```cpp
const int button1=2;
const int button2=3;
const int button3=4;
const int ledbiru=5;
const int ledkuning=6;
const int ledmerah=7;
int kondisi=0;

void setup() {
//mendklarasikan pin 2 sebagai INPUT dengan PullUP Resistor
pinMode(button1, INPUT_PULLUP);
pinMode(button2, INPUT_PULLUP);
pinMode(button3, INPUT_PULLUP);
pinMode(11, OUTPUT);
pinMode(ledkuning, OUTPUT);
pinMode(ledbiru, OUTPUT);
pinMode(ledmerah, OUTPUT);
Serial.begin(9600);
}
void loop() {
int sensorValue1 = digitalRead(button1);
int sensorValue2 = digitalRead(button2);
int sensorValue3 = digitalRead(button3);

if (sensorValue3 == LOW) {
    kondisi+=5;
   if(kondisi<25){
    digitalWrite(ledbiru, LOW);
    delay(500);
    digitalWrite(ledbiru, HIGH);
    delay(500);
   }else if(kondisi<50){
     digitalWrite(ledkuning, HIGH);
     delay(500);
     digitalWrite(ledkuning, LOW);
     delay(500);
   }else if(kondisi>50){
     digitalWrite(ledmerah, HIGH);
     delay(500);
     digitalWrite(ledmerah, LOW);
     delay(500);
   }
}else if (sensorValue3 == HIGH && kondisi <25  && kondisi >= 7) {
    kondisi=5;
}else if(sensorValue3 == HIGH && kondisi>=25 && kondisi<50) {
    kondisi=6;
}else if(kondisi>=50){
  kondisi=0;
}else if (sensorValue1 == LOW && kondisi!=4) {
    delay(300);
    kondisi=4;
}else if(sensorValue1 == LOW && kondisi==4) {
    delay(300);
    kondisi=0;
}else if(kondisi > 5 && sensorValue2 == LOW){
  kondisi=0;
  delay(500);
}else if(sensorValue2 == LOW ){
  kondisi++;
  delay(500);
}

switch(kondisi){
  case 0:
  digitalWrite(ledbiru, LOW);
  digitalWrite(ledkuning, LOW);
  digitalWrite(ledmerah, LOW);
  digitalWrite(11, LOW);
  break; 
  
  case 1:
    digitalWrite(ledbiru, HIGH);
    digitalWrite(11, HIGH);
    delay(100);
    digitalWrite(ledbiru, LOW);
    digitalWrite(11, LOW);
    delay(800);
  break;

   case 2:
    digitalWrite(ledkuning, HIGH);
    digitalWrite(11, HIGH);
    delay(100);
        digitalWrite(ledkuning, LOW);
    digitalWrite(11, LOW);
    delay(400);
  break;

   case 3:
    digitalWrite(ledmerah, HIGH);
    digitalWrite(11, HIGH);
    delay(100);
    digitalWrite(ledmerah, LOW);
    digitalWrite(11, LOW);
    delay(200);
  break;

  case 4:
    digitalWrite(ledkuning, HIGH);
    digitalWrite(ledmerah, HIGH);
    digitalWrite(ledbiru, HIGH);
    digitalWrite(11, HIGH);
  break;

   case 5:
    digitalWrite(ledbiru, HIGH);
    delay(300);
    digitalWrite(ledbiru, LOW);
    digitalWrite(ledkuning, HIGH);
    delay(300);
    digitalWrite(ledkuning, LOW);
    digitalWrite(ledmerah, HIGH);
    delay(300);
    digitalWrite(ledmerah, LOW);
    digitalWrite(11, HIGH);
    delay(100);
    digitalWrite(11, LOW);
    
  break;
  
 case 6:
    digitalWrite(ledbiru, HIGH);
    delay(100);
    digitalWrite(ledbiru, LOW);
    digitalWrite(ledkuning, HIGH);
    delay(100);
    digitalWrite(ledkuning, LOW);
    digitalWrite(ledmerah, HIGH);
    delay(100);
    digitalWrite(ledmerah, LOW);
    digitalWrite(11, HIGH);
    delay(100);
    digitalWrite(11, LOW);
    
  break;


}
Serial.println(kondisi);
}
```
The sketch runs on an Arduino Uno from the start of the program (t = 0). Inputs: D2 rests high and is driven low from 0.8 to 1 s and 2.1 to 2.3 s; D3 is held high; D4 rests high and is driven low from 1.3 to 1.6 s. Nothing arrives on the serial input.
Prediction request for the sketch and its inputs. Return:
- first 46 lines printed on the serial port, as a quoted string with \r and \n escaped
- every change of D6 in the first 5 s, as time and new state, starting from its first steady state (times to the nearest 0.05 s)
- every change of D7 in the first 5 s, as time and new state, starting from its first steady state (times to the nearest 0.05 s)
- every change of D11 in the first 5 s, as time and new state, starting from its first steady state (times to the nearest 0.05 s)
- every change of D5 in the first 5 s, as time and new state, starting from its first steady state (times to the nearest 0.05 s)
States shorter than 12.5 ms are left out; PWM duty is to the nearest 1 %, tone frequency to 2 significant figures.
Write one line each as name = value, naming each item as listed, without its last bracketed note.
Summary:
first 46 lines printed on the serial port, as a quoted string with \r and \n escaped = "0\r\n0\r\n0\r\n0\r\n0\r\n0\r\n0\r\n0\r\n0\r\n0\r\n0\r\n0\r\n0\r\n0\r\n0\r\n0\r\n0\r\n0\r\n0\r\n0\r\n0\r\n0\r\n0\r\n0\r\n0\r\n0\r\n0\r\n0\r\n0\r\n0\r\n0\r\n0\r\n0\r\n0\r\n0\r\n0\r\n0\r\n0\r\n0\r\n0\r\n0\r\n0\r\n0\r\n0\r\n0\r\n0\r\n"
every change of D6 in the first 5 s, as time and new state, starting from its first steady state = 0 s low; 1.1 s high; 2.9 s low; 3.6 s high; 3.9 s low; 4.6 s high; 4.9 s low
every change of D7 in the first 5 s, as time and new state, starting from its first steady state = 0 s low; 1.1 s high; 3.2 s low; 3.9 s high; 4.2 s low; 4.9 s high
every change of D11 in the first 5 s, as time and new state, starting from its first steady state = 0 s low; 1.1 s high; 3.3 s low; 4.2 s high; 4.3 s low
every change of D5 in the first 5 s, as time and new state, starting from its first steady state = 0 s low; 1.1 s high; 1.3 s low; 1.8 s high; 2.6 s low; 3.3 s high; 3.6 s low; 4.3 s high; 4.6 s low
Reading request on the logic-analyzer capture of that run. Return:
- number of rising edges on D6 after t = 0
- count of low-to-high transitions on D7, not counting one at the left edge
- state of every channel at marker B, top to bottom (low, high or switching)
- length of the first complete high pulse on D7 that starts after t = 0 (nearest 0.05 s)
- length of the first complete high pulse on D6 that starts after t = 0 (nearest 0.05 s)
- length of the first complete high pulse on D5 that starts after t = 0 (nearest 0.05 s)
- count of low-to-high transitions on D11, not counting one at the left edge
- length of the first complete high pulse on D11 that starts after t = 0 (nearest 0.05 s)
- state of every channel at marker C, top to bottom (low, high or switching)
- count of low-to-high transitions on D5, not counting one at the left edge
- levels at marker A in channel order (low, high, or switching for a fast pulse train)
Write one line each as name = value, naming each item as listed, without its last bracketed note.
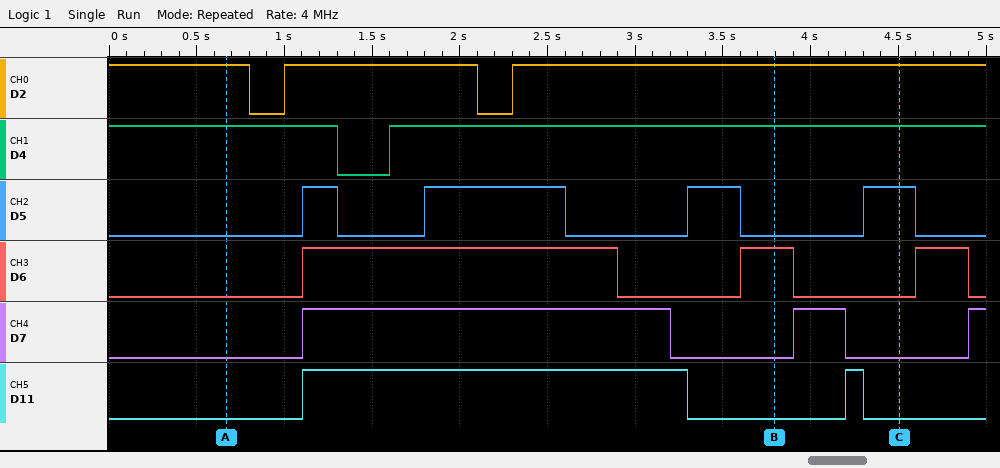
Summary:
number of rising edges on D6 after t = 0 = 3
count of low-to-high transitions on D7, not counting one at the left edge = 3
state of every channel at marker B, top to bottom = D2 high, D4 high, D5 low, D6 high, D7 low, D11 low
length of the first complete high pulse on D7 that starts after t = 0 = 2.10 s
length of the first complete high pulse on D6 that starts after t = 0 = 1.80 s
length of the first complete high pulse on D5 that starts after t = 0 = 0.20 s
count of low-to-high transitions on D11, not counting one at the left edge = 2
length of the first complete high pulse on D11 that starts after t = 0 = 2.20 s
state of every channel at marker C, top to bottom = D2 high, D4 high, D5 high, D6 low, D7 low, D11 low
count of low-to-high transitions on D5, not counting one at the left edge = 4
levels at marker A in channel order = D2 high, D4 high, D5 low, D6 low, D7 low, D11 low
